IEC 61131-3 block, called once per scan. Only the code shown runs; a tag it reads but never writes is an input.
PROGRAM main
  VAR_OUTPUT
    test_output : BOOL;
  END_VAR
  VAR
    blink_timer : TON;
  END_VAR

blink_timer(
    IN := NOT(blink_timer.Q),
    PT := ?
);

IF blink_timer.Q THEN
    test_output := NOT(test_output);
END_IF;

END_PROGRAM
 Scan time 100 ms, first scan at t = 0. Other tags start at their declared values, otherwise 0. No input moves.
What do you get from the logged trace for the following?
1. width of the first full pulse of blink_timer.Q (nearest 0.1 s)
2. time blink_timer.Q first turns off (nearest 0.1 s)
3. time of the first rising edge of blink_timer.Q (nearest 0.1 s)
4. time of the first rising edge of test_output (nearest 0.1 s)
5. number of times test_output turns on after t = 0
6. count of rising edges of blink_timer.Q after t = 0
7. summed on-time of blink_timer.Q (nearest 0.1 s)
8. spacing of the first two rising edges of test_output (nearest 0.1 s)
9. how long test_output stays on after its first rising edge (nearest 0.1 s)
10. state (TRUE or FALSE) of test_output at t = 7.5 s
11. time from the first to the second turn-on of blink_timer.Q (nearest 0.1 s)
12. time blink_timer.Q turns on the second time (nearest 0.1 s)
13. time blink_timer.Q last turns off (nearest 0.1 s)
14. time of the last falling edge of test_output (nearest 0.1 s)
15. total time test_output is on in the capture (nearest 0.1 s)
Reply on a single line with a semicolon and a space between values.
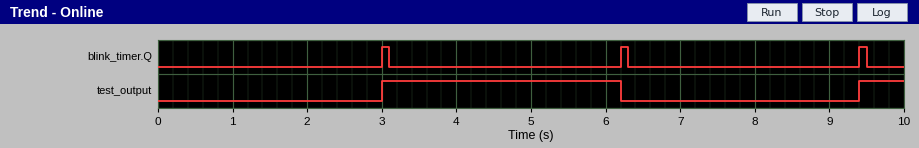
0.1 s; 3.1 s; 3.0 s; 3.0 s; 2; 3; 0.3 s; 6.4 s; 3.2 s; FALSE; 3.2 s; 6.2 s; 9.5 s; 6.2 s; 3.8 s
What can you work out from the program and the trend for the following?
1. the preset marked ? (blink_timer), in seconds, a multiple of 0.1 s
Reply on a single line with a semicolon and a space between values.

3.0 s
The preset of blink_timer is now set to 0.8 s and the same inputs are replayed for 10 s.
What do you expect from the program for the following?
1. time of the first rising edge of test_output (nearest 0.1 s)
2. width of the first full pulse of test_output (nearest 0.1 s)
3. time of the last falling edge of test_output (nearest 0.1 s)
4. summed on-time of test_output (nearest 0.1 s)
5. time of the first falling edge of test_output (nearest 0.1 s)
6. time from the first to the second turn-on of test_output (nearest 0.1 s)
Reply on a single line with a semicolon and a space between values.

0.8 s; 1.0 s; 9.8 s; 5.0 s; 1.8 s; 2.0 s
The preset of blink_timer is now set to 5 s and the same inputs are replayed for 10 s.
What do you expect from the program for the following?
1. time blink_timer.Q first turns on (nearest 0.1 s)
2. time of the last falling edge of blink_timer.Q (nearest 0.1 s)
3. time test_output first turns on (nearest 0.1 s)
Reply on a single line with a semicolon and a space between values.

5.0 s; 5.1 s; 5.0 s
